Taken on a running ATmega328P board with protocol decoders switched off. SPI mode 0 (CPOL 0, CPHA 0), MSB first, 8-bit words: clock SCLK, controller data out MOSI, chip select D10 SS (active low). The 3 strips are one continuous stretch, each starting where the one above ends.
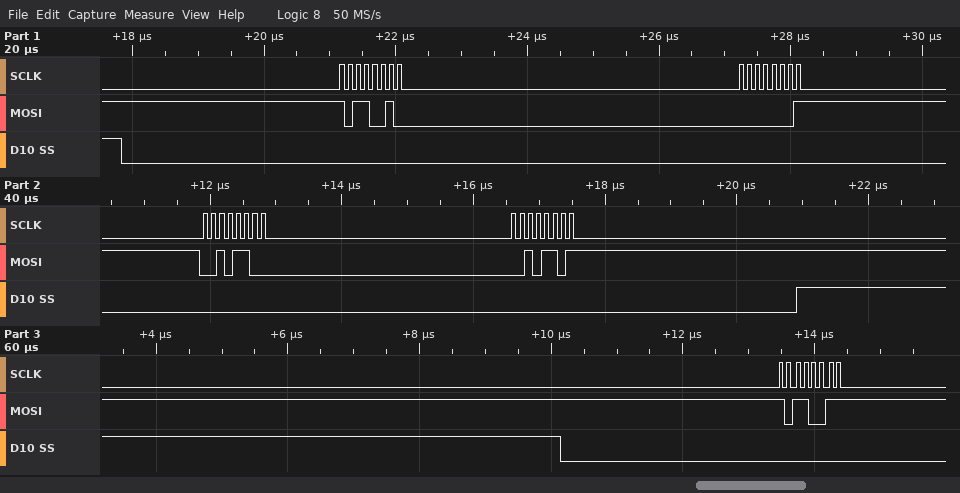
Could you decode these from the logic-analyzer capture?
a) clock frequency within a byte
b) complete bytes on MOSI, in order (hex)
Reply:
8 MHz
B2 01 2C 2D B3
